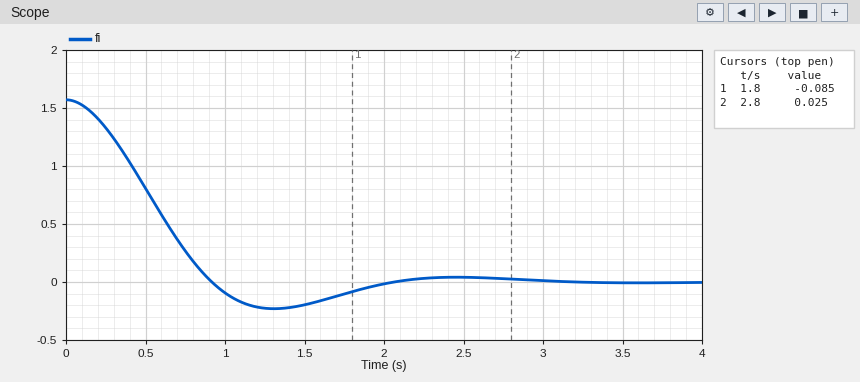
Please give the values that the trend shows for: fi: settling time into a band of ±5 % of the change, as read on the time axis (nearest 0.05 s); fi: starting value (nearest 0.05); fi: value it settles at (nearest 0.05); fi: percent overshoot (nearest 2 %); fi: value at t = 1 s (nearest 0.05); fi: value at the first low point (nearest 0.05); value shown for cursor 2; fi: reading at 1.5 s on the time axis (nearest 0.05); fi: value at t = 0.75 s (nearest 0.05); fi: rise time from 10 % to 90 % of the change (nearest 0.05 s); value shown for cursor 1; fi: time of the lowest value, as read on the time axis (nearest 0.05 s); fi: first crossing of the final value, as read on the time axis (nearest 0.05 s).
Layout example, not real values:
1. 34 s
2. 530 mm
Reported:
1. 1.80 s
2. 1.55
3. 0.00
4. 14 %
5. -0.10
6. -0.25
7. 0.025
8. -0.20
9. 0.25
10. 0.60 s
11. -0.085
12. 1.30 s
13. 0.90 s
